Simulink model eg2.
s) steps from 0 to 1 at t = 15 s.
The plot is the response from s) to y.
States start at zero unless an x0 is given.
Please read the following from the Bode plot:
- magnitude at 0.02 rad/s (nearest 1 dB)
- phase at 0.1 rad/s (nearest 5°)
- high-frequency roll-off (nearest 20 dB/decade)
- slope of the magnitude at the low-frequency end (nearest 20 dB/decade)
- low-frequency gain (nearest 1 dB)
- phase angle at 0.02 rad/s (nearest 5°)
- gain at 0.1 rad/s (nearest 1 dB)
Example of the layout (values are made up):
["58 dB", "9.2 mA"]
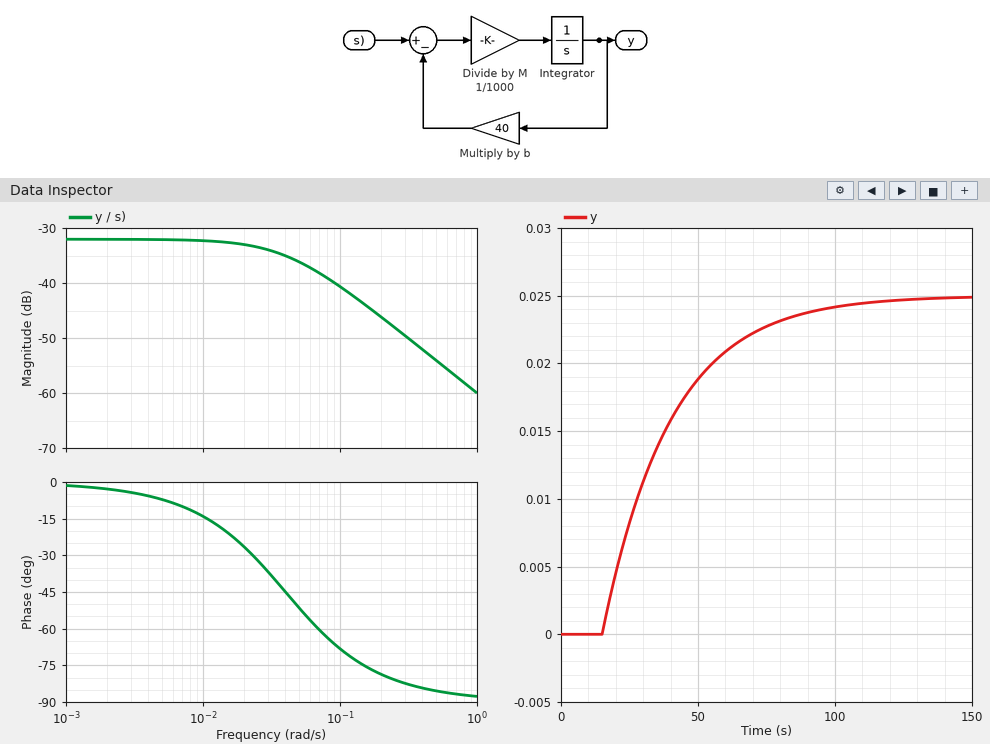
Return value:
["-33 dB", "-70°", "-20 dB/decade", "0 dB/decade", "-32 dB", "-25°", "-41 dB"]
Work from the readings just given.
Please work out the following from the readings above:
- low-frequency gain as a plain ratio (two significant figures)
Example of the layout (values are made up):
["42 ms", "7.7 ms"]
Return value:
["0.025"]
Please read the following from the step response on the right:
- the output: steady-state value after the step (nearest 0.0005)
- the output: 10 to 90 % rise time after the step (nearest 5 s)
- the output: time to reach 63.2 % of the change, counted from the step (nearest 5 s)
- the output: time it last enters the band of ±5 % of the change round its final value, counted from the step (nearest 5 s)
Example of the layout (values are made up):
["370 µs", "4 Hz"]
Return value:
["0.0250", "55 s", "25 s", "75 s"]
